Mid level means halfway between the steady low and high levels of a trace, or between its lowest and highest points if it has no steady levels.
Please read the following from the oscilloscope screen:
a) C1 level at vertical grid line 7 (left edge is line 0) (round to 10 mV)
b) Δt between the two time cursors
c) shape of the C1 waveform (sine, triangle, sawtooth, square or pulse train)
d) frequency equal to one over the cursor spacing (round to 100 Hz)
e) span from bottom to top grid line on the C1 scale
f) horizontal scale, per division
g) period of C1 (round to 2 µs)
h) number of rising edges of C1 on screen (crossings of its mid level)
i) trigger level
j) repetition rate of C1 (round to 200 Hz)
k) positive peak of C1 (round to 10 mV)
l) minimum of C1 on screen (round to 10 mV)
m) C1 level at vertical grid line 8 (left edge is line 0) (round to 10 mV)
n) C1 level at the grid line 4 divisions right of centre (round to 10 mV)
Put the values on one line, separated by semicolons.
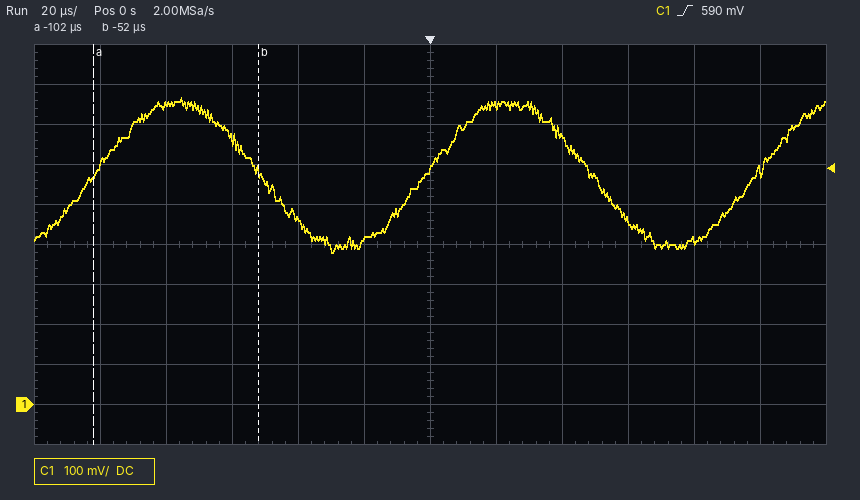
750 mV; 50 µs; sine; 20.0 kHz; 1 V; 20 µs; 100 µs; 3; 590 mV; 10.0 kHz; 770 mV; 380 mV; 670 mV; 410 mV
